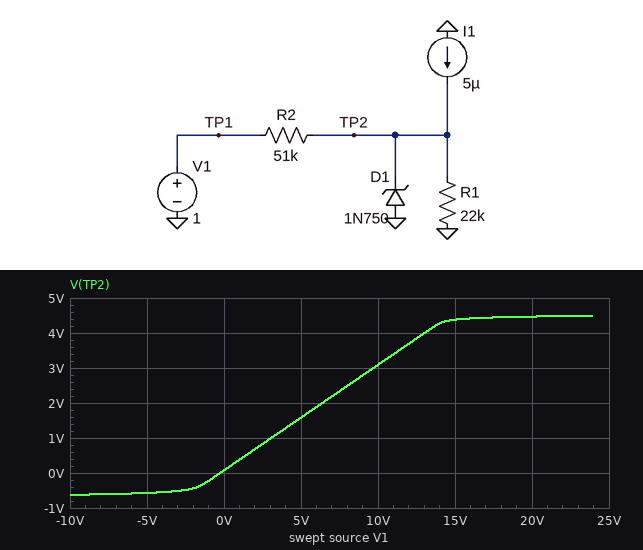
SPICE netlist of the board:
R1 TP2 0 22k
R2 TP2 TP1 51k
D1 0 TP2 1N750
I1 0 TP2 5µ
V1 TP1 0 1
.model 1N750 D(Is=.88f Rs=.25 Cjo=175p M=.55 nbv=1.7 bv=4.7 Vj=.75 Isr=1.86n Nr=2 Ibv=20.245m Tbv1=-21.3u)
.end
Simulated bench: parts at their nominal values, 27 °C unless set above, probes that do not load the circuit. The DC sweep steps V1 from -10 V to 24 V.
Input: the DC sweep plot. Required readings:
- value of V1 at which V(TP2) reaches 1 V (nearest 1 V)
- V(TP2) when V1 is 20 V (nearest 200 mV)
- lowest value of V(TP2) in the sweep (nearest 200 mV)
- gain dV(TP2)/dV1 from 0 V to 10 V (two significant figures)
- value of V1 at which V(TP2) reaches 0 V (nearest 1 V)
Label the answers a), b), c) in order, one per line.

a) 3 V
b) 4.4 V
c) -600 mV
d) 0.30 V/V
e) 0 V
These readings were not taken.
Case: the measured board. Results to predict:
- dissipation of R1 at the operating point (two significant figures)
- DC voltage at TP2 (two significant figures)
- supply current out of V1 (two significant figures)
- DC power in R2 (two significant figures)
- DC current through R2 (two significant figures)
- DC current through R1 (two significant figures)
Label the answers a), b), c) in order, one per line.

a) 6.5 µW
b) 380 mV
c) 12 µA
d) 7.6 µW
e) 12 µA
f) 17 µA
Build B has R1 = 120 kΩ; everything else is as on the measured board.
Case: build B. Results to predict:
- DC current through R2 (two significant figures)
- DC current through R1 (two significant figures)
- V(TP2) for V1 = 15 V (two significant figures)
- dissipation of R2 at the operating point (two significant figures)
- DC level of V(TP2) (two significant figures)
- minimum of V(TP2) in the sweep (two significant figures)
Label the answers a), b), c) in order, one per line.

a) 2.3 µA
b) 7.3 µA
c) 4.5 V
d) 280 nW
e) 880 mV
f) -630 mV
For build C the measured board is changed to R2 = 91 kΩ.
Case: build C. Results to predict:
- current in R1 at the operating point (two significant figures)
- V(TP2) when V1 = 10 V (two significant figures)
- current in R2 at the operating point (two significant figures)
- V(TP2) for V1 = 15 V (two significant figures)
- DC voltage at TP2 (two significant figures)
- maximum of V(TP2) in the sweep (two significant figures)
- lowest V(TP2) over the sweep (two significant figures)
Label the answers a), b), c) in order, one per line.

a) 13 µA
b) 2.0 V
c) 7.9 µA
d) 3.0 V
e) 280 mV
f) 4.4 V
g) -580 mV
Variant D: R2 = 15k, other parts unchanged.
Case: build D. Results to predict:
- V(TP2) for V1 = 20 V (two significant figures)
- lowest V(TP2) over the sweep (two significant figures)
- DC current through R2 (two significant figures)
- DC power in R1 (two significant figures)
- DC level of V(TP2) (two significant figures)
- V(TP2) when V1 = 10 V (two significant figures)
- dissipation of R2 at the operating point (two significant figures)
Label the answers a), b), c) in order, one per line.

a) 4.6 V
b) -680 mV
c) 24 µA
d) 19 µW
e) 640 mV
f) 4.5 V
g) 8.7 µW
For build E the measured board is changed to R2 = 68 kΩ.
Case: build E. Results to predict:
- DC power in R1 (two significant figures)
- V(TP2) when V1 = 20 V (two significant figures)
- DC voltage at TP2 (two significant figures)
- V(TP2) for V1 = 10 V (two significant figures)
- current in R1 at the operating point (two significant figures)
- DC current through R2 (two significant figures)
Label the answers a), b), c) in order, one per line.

a) 4.9 µW
b) 4.4 V
c) 330 mV
d) 2.5 V
e) 15 µA
f) 9.9 µA
